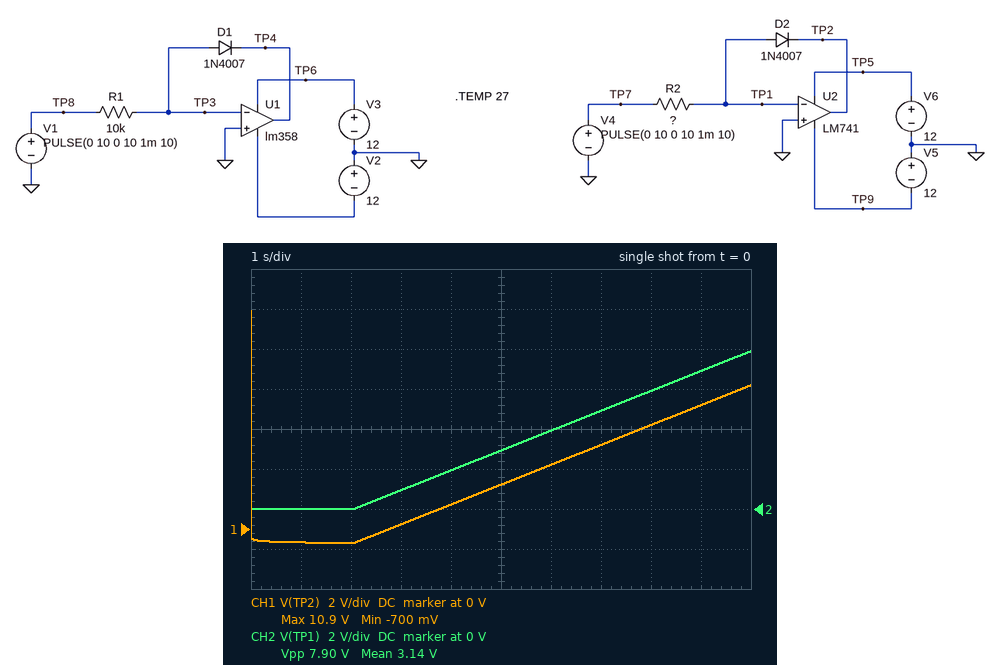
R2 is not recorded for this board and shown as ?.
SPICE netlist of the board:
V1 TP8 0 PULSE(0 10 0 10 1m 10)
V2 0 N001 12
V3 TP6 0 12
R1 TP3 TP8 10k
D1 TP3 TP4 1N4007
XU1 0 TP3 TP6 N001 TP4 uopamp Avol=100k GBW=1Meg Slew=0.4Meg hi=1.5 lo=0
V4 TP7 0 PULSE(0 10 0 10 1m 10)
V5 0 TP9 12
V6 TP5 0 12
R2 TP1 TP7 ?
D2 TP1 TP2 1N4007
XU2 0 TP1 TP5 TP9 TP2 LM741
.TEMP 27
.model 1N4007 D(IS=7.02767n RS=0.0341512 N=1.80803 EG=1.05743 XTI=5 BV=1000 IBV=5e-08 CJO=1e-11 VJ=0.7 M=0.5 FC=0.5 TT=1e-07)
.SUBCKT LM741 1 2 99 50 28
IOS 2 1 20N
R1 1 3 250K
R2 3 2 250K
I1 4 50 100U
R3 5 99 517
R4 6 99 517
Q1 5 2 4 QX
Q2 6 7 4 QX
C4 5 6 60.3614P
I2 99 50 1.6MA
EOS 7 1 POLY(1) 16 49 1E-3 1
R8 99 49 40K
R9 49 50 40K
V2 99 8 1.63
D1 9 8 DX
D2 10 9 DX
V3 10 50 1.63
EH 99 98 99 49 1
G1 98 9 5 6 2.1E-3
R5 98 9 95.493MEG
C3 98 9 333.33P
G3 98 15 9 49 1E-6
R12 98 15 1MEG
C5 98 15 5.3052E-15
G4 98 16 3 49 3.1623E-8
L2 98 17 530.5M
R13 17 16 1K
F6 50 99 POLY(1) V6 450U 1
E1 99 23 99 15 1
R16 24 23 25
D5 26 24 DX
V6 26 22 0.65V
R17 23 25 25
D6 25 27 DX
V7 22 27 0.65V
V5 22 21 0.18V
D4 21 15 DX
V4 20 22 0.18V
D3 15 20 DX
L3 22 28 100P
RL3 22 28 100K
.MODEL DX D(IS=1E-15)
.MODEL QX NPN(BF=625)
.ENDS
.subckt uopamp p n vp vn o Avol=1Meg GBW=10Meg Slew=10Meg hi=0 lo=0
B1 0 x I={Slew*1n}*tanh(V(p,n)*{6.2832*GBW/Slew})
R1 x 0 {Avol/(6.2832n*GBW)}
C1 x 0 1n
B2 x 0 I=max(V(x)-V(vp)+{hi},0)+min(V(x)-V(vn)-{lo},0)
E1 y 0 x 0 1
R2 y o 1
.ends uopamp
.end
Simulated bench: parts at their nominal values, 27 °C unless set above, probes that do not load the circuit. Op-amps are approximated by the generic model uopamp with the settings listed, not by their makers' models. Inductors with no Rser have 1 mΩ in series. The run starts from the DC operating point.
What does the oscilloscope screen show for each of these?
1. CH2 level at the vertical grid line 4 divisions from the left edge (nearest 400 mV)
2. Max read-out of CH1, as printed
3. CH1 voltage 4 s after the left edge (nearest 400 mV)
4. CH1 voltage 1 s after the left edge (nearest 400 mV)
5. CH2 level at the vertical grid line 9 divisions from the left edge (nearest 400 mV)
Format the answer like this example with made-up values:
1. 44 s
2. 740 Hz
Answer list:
1. 2.0 V
2. 10.9 V
3. 1.2 V
4. -800 mV
5. 6.8 V
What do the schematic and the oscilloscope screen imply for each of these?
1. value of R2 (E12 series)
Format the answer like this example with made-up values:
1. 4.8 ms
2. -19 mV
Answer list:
1. 82 Ω
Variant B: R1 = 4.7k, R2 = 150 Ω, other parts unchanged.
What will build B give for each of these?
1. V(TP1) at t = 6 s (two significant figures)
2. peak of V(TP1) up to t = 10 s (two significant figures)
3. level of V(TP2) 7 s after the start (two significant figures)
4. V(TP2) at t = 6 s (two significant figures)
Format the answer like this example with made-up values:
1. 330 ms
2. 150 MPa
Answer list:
1. 2.2 V
2. 6.2 V
3. 2.5 V
4. 1.5 V
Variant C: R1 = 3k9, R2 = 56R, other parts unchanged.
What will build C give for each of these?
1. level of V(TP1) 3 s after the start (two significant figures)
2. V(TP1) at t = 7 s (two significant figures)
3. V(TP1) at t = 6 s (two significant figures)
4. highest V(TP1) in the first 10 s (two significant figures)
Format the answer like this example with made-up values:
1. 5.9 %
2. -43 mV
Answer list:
1. 1.6 V
2. 5.6 V
3. 4.6 V
4. 8.6 V
